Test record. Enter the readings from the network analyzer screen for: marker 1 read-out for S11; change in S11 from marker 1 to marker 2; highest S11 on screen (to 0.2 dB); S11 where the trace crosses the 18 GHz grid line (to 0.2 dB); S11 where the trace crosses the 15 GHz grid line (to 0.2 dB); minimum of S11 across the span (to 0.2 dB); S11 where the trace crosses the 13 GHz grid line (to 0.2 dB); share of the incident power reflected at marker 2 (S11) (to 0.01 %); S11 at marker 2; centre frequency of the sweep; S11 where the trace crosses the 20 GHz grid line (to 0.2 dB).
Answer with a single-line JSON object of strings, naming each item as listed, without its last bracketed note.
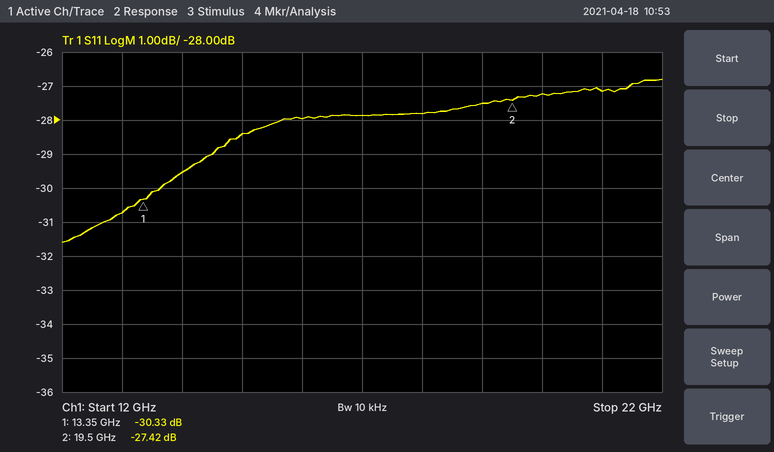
{"marker 1 read-out for S11": "-30.33 dB", "change in S11 from marker 1 to marker 2": "2.91 dB", "highest S11 on screen": "-26.8 dB", "S11 where the trace crosses the 18 GHz grid line": "-27.8 dB", "S11 where the trace crosses the 15 GHz grid line": "-28.4 dB", "minimum of S11 across the span": "-31.6 dB", "S11 where the trace crosses the 13 GHz grid line": "-30.8 dB", "share of the incident power reflected at marker 2 (S11)": "0.18 %", "S11 at marker 2": "-27.42 dB", "centre frequency of the sweep": "17 GHz", "S11 where the trace crosses the 20 GHz grid line": "-27.2 dB"}
